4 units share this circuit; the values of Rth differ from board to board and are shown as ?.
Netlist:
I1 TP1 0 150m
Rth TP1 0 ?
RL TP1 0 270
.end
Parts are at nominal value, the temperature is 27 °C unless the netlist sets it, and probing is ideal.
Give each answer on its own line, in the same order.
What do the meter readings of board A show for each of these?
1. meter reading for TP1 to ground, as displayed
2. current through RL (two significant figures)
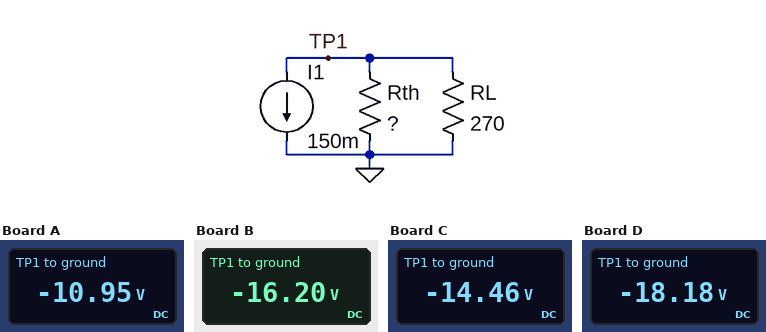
-10.95 V
41 mA
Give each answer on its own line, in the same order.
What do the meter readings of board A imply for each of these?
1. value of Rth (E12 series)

100 Ω
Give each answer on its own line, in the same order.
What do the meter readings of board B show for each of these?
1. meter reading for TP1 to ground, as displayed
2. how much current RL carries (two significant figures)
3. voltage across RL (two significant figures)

-16.20 V
60 mA
16 V
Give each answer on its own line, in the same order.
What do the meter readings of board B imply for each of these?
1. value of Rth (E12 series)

180 Ω
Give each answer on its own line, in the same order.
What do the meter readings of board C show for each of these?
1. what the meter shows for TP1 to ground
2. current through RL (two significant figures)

-14.46 V
54 mA
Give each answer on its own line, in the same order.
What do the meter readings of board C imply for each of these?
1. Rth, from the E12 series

150 Ω
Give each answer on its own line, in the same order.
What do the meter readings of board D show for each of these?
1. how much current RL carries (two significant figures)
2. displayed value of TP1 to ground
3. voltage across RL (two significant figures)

67 mA
-18.18 V
18 V
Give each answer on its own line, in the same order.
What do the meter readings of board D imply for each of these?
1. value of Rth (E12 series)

220 Ω
